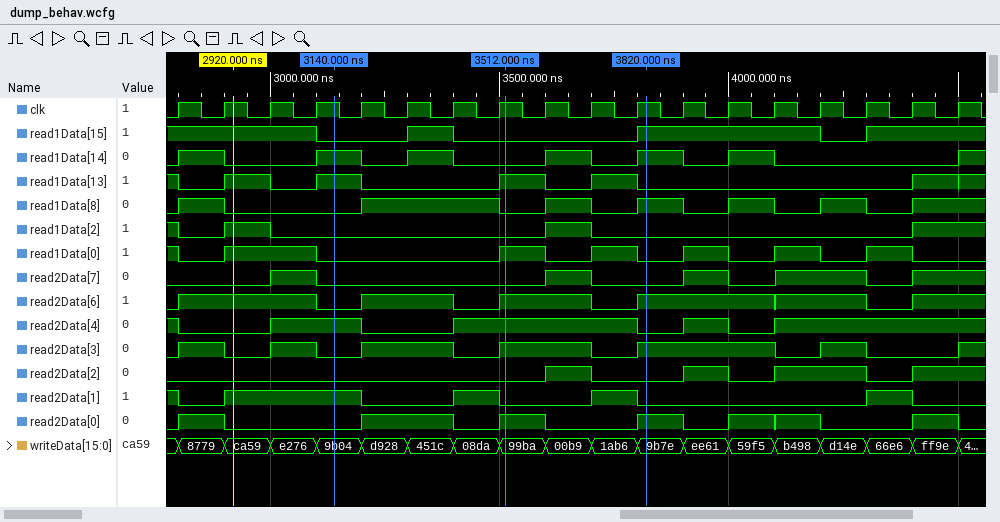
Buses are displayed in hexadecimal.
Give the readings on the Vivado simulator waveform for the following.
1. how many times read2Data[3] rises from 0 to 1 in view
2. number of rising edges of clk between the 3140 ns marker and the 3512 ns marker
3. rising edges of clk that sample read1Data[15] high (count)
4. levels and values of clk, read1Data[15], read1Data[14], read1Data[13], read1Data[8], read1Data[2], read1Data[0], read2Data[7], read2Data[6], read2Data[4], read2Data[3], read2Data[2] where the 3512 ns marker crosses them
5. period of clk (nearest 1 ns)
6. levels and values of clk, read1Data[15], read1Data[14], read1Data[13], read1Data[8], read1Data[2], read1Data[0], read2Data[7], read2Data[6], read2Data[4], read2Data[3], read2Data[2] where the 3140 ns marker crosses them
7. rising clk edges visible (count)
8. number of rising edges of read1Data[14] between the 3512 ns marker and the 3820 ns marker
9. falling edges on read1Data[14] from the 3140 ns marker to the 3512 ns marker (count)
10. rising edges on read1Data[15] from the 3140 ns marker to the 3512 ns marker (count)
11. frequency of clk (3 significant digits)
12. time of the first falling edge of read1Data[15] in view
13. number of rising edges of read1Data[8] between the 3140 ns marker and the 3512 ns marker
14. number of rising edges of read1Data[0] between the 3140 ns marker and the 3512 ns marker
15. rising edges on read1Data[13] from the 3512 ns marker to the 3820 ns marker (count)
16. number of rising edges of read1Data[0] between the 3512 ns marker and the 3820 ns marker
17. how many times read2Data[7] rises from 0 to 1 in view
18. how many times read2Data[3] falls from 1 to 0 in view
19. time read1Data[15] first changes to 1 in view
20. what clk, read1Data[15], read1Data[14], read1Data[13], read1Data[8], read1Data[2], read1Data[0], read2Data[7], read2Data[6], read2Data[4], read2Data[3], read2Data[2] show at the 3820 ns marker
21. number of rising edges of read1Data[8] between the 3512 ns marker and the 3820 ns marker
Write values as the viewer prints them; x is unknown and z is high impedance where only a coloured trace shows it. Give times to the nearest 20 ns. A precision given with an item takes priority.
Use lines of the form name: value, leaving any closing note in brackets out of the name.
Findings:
how many times read2Data[3] rises from 0 to 1 in view: 7
number of rising edges of clk between the 3140 ns marker and the 3512 ns marker: 4
rising edges of clk that sample read1Data[15] high: 11
levels and values of clk, read1Data[15], read1Data[14], read1Data[13], read1Data[8], read1Data[2], read1Data[0], read2Data[7], read2Data[6], read2Data[4], read2Data[3], read2Data[2] where the 3512 ns marker crosses them: clk=1, read1Data[15]=0, read1Data[14]=0, read1Data[13]=1, read1Data[8]=0, read1Data[2]=0, read1Data[0]=1, read2Data[7]=0, read2Data[6]=1, read2Data[4]=1, read2Data[3]=1, read2Data[2]=0
period of clk: 100 ns
levels and values of clk, read1Data[15], read1Data[14], read1Data[13], read1Data[8], read1Data[2], read1Data[0], read2Data[7], read2Data[6], read2Data[4], read2Data[3], read2Data[2] where the 3140 ns marker crosses them: clk=1, read1Data[15]=0, read1Data[14]=1, read1Data[13]=1, read1Data[8]=0, read1Data[2]=0, read1Data[0]=0, read2Data[7]=0, read2Data[6]=0, read2Data[4]=1, read2Data[3]=0, read2Data[2]=0
rising clk edges visible: 18
number of rising edges of read1Data[14] between the 3512 ns marker and the 3820 ns marker: 2
falling edges on read1Data[14] from the 3140 ns marker to the 3512 ns marker: 2
rising edges on read1Data[15] from the 3140 ns marker to the 3512 ns marker: 1
frequency of clk: 10.0 MHz
time of the first falling edge of read1Data[15] in view: 3100 ns
number of rising edges of read1Data[8] between the 3140 ns marker and the 3512 ns marker: 1
number of rising edges of read1Data[0] between the 3140 ns marker and the 3512 ns marker: 1
rising edges on read1Data[13] from the 3512 ns marker to the 3820 ns marker: 1
number of rising edges of read1Data[0] between the 3512 ns marker and the 3820 ns marker: 1
how many times read2Data[7] rises from 0 to 1 in view: 5
how many times read2Data[3] falls from 1 to 0 in view: 6
time read1Data[15] first changes to 1 in view: 3300 ns
what clk, read1Data[15], read1Data[14], read1Data[13], read1Data[8], read1Data[2], read1Data[0], read2Data[7], read2Data[6], read2Data[4], read2Data[3], read2Data[2] show at the 3820 ns marker: clk=1, read1Data[15]=1, read1Data[14]=1, read1Data[13]=0, read1Data[8]=1, read1Data[2]=0, read1Data[0]=0, read2Data[7]=0, read2Data[6]=1, read2Data[4]=0, read2Data[3]=1, read2Data[2]=0
number of rising edges of read1Data[8] between the 3512 ns marker and the 3820 ns marker: 2
